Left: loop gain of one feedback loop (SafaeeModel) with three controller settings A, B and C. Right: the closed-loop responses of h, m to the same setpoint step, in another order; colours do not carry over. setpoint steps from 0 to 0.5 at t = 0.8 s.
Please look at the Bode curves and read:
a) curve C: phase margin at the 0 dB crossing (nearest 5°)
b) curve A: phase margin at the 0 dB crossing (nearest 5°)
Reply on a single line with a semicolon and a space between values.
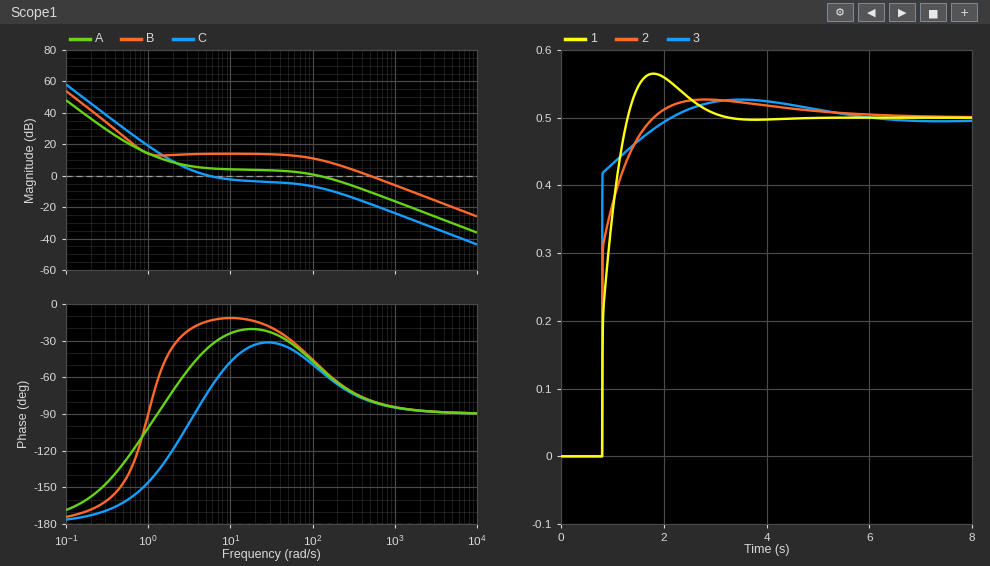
110°; 130°
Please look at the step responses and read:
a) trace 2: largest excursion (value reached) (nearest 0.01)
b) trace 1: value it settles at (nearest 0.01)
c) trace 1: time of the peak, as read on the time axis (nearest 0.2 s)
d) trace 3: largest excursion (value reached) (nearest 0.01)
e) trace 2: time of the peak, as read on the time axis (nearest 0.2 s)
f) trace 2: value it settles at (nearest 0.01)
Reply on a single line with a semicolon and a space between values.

0.53; 0.50; 1.8 s; 0.53; 2.8 s; 0.50
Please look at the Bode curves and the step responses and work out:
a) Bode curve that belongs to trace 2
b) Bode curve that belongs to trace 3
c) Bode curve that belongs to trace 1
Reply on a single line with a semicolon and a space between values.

A; B; C
